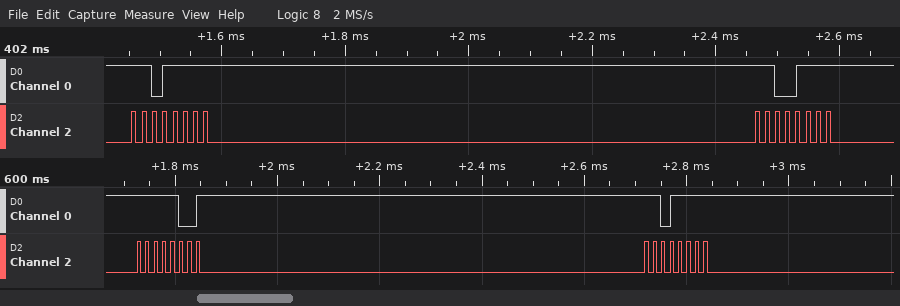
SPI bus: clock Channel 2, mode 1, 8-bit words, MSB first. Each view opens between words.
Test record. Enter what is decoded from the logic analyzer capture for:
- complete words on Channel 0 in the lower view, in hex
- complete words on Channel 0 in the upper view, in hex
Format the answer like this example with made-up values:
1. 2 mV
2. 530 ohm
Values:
1. F9, DF
2. DF, CF
